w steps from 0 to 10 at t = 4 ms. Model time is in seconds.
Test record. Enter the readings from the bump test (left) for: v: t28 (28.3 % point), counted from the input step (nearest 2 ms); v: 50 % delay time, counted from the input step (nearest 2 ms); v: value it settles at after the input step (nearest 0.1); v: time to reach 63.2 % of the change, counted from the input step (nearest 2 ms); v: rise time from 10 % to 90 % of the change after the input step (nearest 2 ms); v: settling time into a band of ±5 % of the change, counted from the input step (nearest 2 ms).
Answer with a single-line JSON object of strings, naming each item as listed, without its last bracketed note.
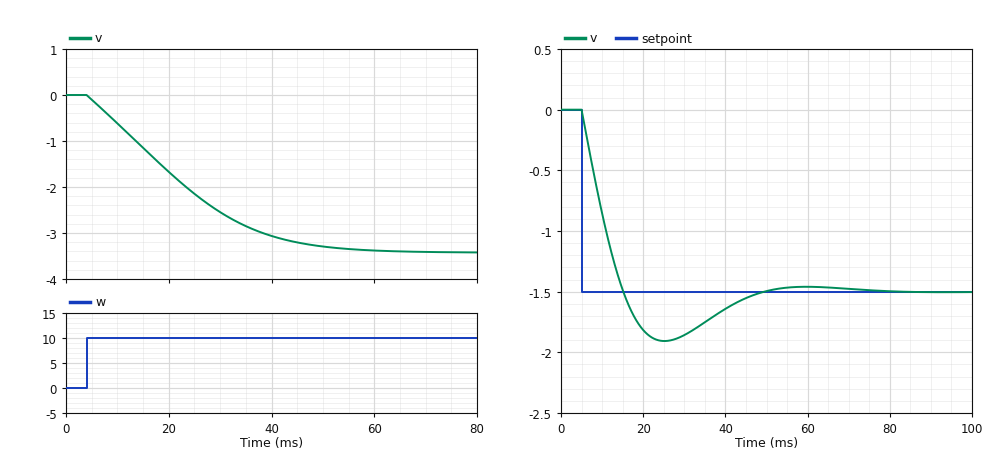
{"v: t28 (28.3 % point), counted from the input step": "10 ms", "v: 50 % delay time, counted from the input step": "16 ms", "v: value it settles at after the input step": "-3.4", "v: time to reach 63.2 % of the change, counted from the input step": "22 ms", "v: rise time from 10 % to 90 % of the change after the input step": "34 ms", "v: settling time into a band of ±5 % of the change, counted from the input step": "44 ms"}
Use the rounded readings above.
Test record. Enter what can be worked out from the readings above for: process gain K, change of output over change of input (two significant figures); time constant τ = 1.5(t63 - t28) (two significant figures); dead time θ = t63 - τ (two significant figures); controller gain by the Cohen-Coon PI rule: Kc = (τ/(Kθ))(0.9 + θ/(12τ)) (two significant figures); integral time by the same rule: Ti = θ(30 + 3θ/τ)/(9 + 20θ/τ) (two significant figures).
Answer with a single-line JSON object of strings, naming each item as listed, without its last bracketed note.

{"process gain K, change of output over change of input": "-0.34", "time constant τ = 1.5(t63 - t28)": "18 ms", "dead time θ = t63 - τ": "4.0 ms", "controller gain by the Cohen-Coon PI rule: Kc = (τ/(Kθ))(0.9 + θ/(12τ))": "-12", "integral time by the same rule: Ti = θ(30 + 3θ/τ)/(9 + 20θ/τ)": "9.1 ms"}
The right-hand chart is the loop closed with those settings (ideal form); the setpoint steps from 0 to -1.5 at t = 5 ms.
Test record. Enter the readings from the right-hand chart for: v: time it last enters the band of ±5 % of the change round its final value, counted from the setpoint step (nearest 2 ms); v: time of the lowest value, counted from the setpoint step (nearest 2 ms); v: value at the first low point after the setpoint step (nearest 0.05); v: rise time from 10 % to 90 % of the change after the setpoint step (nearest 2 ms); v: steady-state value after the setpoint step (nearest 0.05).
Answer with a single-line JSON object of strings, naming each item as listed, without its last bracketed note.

{"v: time it last enters the band of ±5 % of the change round its final value, counted from the setpoint step": "38 ms", "v: time of the lowest value, counted from the setpoint step": "20 ms", "v: value at the first low point after the setpoint step": "-1.90", "v: rise time from 10 % to 90 % of the change after the setpoint step": "8 ms", "v: steady-state value after the setpoint step": "-1.50"}
